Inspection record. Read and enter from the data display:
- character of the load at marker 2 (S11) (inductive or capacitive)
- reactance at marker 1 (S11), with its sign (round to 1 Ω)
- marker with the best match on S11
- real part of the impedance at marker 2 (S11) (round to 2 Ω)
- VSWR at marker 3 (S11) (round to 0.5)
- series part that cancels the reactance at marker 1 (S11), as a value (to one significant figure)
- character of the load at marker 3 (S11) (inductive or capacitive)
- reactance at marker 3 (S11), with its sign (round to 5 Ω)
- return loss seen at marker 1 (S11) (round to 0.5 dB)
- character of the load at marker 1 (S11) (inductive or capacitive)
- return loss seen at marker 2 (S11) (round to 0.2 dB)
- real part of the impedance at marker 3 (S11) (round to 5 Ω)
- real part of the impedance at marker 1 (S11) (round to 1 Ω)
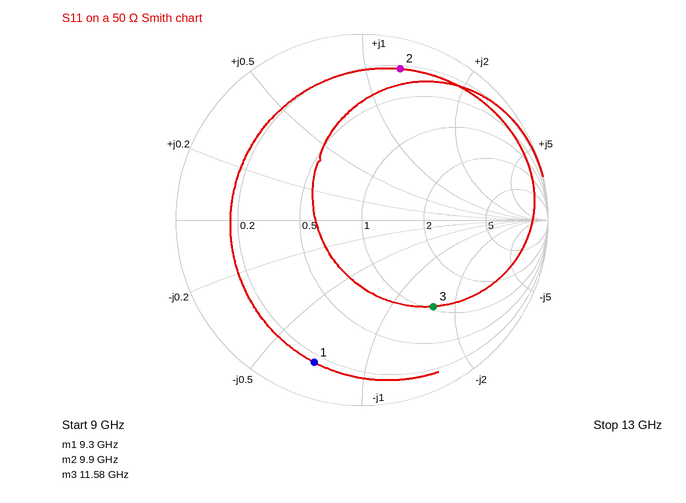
inductive
-35 Ω
marker 3
12 Ω
4.0
600 pH
capacitive
-80 Ω
2.0 dB
capacitive
1.6 dB
55 Ω
8 Ω
